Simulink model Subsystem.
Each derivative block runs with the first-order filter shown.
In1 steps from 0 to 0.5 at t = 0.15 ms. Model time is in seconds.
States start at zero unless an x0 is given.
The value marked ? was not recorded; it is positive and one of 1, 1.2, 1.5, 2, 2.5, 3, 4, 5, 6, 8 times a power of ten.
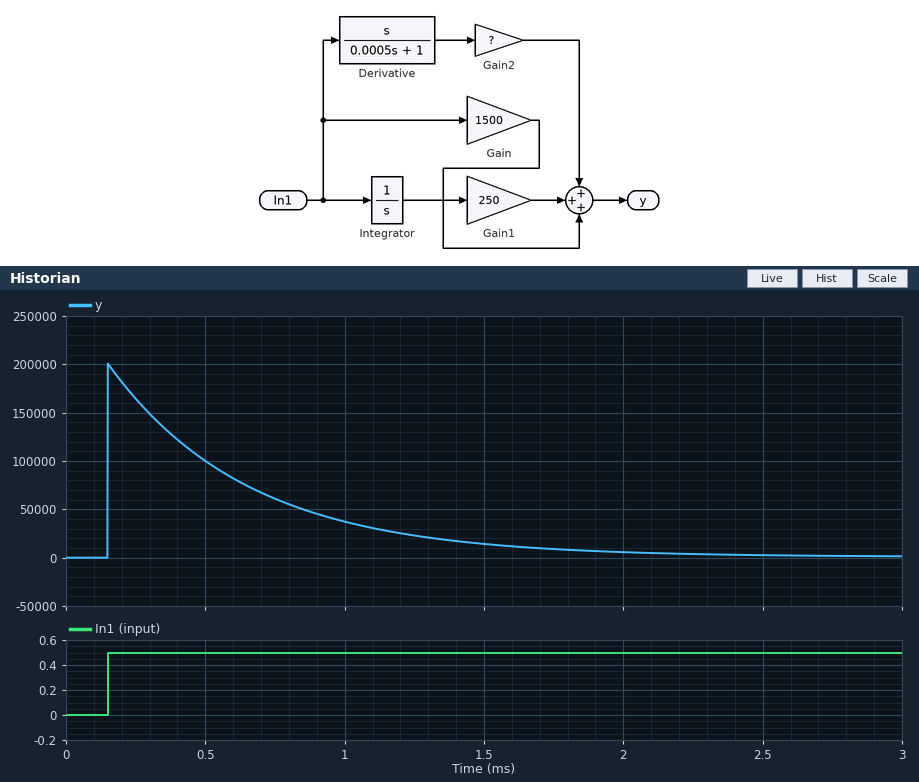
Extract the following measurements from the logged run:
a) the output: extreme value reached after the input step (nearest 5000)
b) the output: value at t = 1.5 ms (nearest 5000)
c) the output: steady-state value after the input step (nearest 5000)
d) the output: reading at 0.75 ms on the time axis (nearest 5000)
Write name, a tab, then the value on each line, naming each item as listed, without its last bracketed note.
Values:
the output: extreme value reached after the input step	200000
the output: value at t = 1.5 ms	15000
the output: steady-state value after the input step	0
the output: reading at 0.75 ms on the time axis	60000
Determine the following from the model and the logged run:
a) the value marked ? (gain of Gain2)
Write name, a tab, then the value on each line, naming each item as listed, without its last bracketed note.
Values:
the value marked ?	200
